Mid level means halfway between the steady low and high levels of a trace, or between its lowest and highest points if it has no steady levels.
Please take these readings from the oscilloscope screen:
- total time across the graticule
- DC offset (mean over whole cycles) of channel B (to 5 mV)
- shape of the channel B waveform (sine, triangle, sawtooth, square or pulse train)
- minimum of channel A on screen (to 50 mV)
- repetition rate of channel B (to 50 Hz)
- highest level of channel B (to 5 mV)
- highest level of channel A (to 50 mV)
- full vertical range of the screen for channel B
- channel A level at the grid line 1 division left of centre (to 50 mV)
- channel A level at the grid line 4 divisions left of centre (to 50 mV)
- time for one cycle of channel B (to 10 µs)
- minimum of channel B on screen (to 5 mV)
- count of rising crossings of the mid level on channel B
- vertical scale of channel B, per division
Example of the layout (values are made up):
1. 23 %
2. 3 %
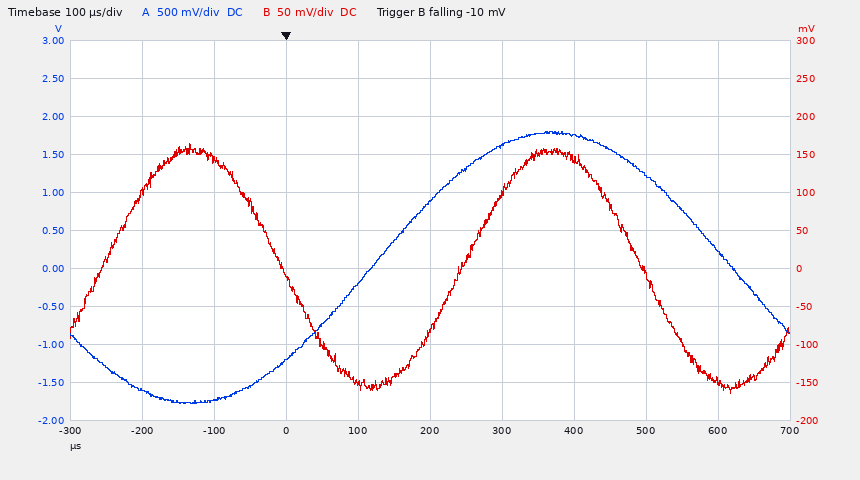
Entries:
1. 1 ms
2. 0 mV
3. sine
4. -1.80 V
5. 2.00 kHz
6. 165 mV
7. 1.80 V
8. 500 mV
9. -200 mV
10. -1.60 V
11. 500 µs
12. -165 mV
13. 2
14. 50 mV
